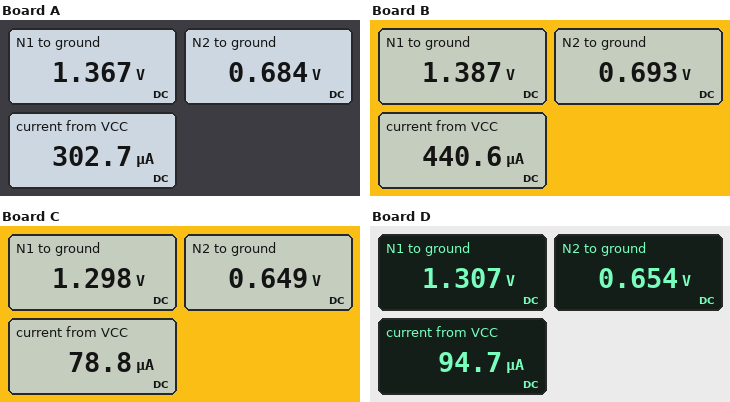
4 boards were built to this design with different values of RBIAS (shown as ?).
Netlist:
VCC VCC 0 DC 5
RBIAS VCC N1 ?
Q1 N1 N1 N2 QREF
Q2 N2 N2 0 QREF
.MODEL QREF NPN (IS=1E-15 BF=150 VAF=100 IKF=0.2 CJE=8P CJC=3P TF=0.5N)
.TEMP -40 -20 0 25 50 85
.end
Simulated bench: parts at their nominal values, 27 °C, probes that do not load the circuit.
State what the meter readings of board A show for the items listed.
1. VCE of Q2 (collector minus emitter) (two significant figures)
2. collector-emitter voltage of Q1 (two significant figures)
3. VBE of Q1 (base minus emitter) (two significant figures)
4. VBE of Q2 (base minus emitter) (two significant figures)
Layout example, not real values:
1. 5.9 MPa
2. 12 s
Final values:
1. 680 mV
2. 680 mV
3. 680 mV
4. 680 mV
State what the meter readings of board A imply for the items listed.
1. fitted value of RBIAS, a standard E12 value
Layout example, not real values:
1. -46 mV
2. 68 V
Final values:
1. 12 kΩ
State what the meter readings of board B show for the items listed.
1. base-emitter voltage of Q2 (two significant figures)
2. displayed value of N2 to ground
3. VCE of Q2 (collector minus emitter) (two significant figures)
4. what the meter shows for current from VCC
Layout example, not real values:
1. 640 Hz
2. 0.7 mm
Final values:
1. 690 mV
2. 0.693 V
3. 690 mV
4. 440.6 µA
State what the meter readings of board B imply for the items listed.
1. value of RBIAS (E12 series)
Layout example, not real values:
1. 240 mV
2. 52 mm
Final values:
1. 8.2 kΩ
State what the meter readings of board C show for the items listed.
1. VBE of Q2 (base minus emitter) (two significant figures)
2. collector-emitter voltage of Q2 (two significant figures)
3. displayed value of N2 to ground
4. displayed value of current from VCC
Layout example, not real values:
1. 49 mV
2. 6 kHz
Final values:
1. 650 mV
2. 650 mV
3. 0.649 V
4. 78.8 µA
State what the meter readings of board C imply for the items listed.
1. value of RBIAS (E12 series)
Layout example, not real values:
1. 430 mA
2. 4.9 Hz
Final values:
1. 47 kΩ
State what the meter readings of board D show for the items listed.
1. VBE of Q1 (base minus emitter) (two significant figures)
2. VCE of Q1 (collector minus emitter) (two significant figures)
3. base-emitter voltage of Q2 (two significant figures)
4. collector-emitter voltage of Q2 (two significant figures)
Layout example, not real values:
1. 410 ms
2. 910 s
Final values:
1. 650 mV
2. 650 mV
3. 650 mV
4. 650 mV
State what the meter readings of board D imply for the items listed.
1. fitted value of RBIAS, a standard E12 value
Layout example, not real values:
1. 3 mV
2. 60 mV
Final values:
1. 39 kΩ
